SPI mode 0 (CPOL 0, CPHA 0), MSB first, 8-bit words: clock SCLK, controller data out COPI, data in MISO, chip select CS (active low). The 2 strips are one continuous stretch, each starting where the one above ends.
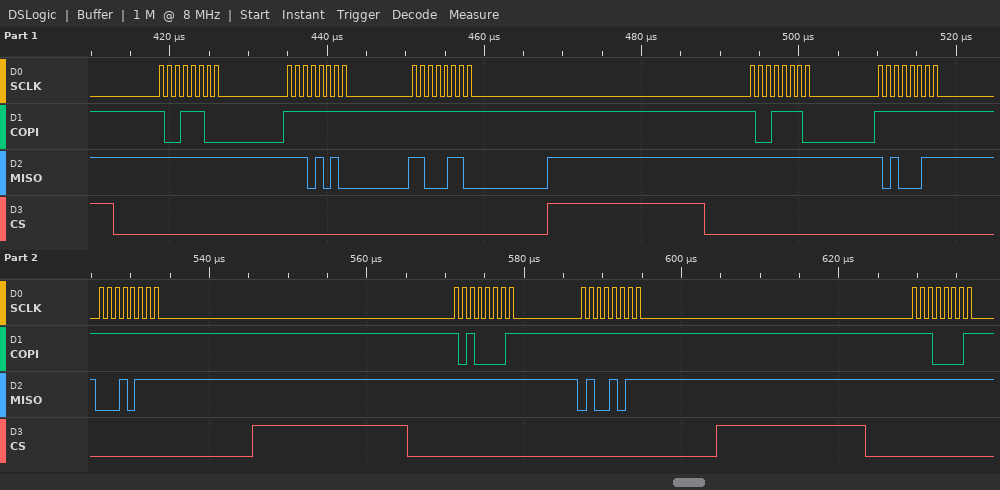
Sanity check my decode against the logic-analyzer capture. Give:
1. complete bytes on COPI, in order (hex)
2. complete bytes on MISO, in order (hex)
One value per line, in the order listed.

9C FF FF 9E FF FF A1 FF E1
FF EA C6 FF A3 17 FF 4B FF
